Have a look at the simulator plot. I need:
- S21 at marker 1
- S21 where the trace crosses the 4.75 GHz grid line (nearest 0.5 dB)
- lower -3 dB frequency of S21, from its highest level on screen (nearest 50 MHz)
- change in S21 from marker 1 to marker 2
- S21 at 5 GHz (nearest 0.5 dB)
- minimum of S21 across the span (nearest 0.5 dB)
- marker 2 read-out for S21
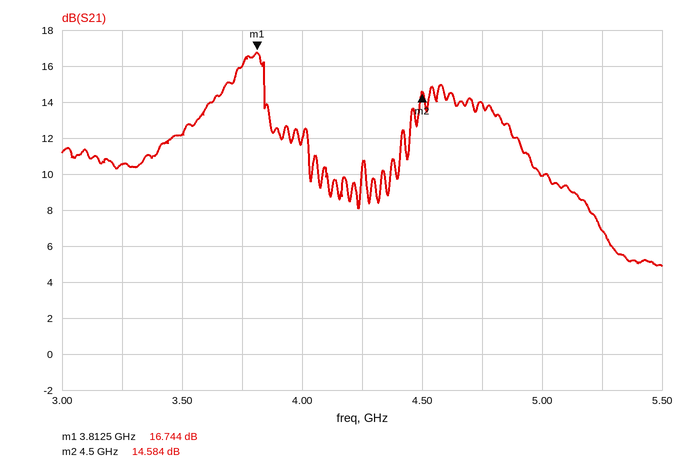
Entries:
16.744 dB
14.0 dB
3.60 GHz
-2.160 dB
10.0 dB
5.0 dB
14.584 dB
